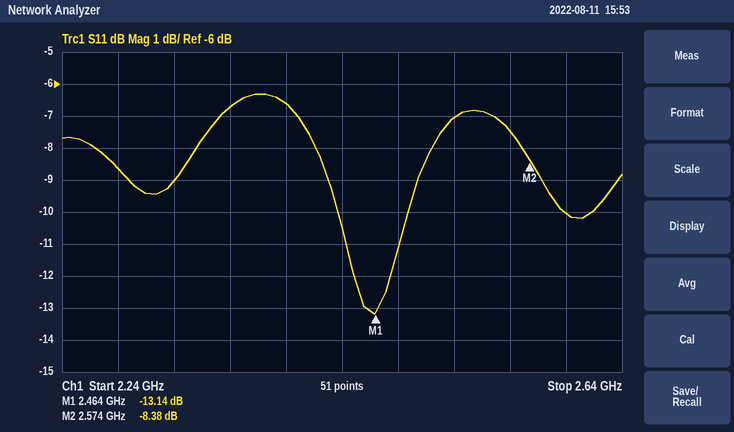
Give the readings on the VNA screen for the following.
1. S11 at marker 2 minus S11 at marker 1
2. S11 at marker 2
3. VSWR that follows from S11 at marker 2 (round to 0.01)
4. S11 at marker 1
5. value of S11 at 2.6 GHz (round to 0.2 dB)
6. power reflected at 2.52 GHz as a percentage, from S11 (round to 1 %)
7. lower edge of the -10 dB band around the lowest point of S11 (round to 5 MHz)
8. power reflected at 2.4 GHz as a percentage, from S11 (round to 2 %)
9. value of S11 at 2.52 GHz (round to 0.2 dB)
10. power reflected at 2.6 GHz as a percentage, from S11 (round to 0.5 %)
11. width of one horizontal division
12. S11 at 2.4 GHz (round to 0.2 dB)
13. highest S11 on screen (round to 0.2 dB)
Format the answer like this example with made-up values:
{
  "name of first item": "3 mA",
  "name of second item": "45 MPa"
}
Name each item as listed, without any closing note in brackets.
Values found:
{
  "S11 at marker 2 minus S11 at marker 1": "4.76 dB",
  "S11 at marker 2": "-8.38 dB",
  "VSWR that follows from S11 at marker 2": "2.23",
  "S11 at marker 1": "-13.14 dB",
  "value of S11 at 2.6 GHz": "-10.0 dB",
  "power reflected at 2.52 GHz as a percentage, from S11": "20 %",
  "lower edge of the -10 dB band around the lowest point of S11": "2.435 GHz",
  "power reflected at 2.4 GHz as a percentage, from S11": "22 %",
  "value of S11 at 2.52 GHz": "-7.0 dB",
  "power reflected at 2.6 GHz as a percentage, from S11": "10.0 %",
  "width of one horizontal division": "40 MHz",
  "S11 at 2.4 GHz": "-6.6 dB",
  "highest S11 on screen": "-6.4 dB"
}
